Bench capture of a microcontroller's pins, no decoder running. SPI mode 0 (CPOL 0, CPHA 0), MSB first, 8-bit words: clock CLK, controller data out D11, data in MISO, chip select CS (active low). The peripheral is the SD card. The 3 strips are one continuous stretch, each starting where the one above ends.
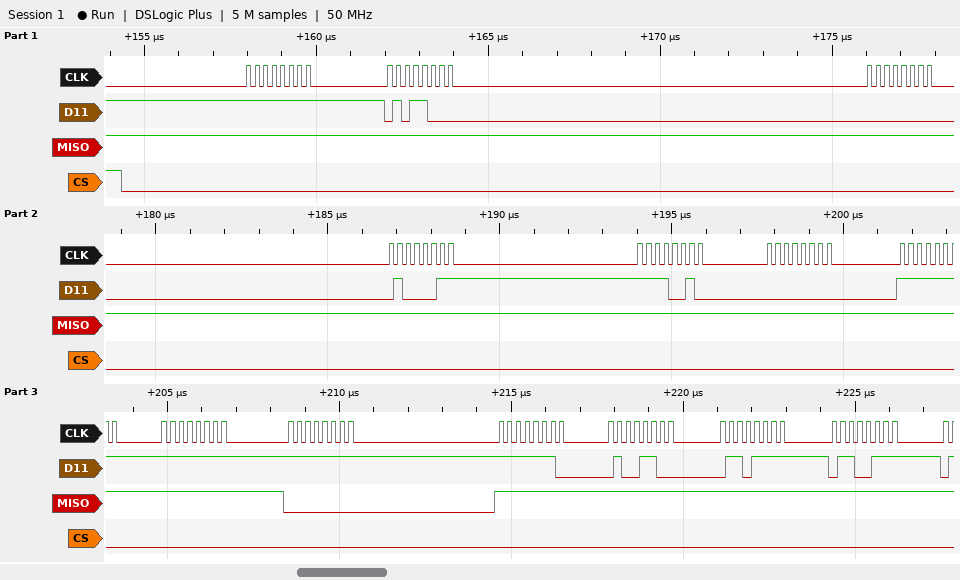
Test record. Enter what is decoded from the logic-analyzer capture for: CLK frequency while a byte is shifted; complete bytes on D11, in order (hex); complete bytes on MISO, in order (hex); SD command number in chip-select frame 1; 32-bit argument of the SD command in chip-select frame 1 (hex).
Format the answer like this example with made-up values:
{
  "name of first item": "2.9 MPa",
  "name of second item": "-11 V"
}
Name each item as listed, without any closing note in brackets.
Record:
{
  "CLK frequency while a byte is shifted": "4 MHz",
  "complete bytes on D11, in order": "FF 58 00 43 F2 00 FF FF FF FE 4C 6F 67",
  "complete bytes on MISO, in order": "FF FF FF FF FF FF FF FF 00 FF FF FF FF",
  "SD command number in chip-select frame 1": "CMD24",
  "32-bit argument of the SD command in chip-select frame 1": "0x0043F200"
}
